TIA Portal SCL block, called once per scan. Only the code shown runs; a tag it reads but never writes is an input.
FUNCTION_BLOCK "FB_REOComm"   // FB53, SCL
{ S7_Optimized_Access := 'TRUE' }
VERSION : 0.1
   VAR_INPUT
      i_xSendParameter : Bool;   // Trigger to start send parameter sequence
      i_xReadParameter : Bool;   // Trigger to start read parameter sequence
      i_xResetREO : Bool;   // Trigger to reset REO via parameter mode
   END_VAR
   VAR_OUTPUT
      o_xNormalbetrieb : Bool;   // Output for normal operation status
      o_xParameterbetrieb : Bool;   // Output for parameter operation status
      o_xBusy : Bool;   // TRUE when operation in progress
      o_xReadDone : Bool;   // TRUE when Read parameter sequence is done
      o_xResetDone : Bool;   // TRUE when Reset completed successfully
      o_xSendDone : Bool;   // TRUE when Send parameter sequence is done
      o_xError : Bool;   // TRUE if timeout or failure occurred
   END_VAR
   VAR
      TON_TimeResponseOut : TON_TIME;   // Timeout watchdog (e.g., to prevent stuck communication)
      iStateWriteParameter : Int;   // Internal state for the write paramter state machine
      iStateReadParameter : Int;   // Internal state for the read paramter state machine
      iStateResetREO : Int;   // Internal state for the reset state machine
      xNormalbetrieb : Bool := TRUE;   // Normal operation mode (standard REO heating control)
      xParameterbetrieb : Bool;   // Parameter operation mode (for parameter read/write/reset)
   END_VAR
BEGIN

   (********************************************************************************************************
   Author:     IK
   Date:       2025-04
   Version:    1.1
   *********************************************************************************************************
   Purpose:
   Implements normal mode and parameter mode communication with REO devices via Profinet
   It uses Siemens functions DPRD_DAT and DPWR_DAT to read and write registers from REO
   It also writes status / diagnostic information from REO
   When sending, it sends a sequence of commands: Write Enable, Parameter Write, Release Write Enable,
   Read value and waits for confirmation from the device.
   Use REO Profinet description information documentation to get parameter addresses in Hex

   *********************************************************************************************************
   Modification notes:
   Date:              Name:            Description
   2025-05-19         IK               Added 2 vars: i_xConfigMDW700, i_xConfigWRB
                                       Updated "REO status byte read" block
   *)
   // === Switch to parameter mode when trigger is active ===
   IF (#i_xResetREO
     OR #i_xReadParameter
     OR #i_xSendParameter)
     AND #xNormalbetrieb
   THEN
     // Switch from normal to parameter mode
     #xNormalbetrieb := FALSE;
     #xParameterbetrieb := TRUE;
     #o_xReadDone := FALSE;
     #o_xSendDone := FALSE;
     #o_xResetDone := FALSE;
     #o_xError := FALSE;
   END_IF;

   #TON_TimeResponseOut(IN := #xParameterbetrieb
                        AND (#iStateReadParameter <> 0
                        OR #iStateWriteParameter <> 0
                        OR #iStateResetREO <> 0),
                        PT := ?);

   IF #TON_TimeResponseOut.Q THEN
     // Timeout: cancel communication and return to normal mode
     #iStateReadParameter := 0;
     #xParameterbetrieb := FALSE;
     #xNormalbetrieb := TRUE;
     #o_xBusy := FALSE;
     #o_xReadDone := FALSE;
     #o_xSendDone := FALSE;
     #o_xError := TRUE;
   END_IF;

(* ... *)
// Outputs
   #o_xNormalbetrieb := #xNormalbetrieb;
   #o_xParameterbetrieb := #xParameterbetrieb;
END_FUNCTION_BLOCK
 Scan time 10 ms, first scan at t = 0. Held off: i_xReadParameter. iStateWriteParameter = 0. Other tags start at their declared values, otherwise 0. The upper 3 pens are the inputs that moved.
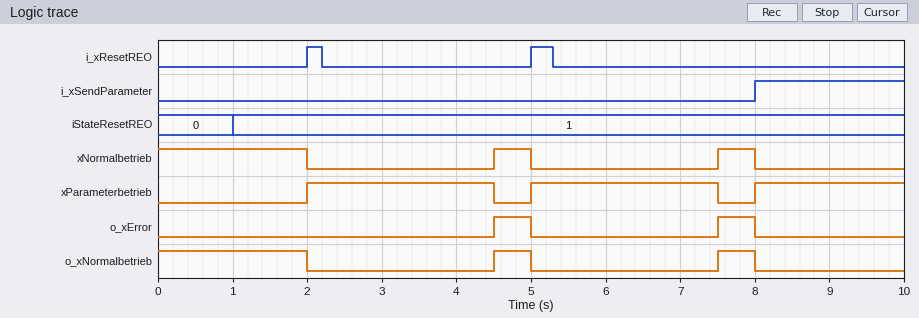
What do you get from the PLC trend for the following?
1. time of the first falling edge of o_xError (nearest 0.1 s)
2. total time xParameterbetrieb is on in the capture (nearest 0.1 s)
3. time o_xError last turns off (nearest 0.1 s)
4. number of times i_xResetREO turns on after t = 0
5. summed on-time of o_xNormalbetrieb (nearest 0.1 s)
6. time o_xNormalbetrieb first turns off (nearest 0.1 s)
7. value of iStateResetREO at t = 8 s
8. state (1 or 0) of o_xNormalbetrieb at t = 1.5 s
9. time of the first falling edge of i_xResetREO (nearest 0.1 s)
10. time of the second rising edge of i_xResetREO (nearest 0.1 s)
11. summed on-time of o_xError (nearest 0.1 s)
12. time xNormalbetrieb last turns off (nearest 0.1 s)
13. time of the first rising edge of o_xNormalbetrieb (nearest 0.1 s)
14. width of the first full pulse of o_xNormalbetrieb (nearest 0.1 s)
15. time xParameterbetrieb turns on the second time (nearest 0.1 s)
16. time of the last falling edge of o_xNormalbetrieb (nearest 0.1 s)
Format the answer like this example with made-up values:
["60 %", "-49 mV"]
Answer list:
["5.0 s", "7.0 s", "8.0 s", "2", "3.0 s", "2.0 s", "1", "1", "2.2 s", "5.0 s", "1.0 s", "8.0 s", "4.5 s", "0.5 s", "5.0 s", "8.0 s"]
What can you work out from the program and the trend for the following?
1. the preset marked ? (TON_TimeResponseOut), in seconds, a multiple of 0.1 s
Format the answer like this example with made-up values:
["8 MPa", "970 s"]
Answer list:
["2.5 s"]
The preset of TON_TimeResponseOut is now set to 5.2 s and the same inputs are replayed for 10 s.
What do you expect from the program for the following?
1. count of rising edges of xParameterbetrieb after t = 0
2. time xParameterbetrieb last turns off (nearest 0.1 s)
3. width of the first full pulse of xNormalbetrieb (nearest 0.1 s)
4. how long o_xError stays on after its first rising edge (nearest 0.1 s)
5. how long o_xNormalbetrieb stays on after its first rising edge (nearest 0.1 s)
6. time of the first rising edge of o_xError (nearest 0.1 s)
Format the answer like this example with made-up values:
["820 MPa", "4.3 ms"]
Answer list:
["2", "7.2 s", "0.8 s", "0.8 s", "0.8 s", "7.2 s"]
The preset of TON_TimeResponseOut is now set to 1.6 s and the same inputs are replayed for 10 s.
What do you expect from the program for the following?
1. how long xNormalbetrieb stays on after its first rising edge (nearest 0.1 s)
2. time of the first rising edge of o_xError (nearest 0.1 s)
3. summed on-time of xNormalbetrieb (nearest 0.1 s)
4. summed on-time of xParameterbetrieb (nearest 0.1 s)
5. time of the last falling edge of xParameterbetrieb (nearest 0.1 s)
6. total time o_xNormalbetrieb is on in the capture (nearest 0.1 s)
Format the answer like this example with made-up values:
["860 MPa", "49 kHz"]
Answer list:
["1.4 s", "3.6 s", "5.2 s", "4.8 s", "9.6 s", "5.2 s"]
